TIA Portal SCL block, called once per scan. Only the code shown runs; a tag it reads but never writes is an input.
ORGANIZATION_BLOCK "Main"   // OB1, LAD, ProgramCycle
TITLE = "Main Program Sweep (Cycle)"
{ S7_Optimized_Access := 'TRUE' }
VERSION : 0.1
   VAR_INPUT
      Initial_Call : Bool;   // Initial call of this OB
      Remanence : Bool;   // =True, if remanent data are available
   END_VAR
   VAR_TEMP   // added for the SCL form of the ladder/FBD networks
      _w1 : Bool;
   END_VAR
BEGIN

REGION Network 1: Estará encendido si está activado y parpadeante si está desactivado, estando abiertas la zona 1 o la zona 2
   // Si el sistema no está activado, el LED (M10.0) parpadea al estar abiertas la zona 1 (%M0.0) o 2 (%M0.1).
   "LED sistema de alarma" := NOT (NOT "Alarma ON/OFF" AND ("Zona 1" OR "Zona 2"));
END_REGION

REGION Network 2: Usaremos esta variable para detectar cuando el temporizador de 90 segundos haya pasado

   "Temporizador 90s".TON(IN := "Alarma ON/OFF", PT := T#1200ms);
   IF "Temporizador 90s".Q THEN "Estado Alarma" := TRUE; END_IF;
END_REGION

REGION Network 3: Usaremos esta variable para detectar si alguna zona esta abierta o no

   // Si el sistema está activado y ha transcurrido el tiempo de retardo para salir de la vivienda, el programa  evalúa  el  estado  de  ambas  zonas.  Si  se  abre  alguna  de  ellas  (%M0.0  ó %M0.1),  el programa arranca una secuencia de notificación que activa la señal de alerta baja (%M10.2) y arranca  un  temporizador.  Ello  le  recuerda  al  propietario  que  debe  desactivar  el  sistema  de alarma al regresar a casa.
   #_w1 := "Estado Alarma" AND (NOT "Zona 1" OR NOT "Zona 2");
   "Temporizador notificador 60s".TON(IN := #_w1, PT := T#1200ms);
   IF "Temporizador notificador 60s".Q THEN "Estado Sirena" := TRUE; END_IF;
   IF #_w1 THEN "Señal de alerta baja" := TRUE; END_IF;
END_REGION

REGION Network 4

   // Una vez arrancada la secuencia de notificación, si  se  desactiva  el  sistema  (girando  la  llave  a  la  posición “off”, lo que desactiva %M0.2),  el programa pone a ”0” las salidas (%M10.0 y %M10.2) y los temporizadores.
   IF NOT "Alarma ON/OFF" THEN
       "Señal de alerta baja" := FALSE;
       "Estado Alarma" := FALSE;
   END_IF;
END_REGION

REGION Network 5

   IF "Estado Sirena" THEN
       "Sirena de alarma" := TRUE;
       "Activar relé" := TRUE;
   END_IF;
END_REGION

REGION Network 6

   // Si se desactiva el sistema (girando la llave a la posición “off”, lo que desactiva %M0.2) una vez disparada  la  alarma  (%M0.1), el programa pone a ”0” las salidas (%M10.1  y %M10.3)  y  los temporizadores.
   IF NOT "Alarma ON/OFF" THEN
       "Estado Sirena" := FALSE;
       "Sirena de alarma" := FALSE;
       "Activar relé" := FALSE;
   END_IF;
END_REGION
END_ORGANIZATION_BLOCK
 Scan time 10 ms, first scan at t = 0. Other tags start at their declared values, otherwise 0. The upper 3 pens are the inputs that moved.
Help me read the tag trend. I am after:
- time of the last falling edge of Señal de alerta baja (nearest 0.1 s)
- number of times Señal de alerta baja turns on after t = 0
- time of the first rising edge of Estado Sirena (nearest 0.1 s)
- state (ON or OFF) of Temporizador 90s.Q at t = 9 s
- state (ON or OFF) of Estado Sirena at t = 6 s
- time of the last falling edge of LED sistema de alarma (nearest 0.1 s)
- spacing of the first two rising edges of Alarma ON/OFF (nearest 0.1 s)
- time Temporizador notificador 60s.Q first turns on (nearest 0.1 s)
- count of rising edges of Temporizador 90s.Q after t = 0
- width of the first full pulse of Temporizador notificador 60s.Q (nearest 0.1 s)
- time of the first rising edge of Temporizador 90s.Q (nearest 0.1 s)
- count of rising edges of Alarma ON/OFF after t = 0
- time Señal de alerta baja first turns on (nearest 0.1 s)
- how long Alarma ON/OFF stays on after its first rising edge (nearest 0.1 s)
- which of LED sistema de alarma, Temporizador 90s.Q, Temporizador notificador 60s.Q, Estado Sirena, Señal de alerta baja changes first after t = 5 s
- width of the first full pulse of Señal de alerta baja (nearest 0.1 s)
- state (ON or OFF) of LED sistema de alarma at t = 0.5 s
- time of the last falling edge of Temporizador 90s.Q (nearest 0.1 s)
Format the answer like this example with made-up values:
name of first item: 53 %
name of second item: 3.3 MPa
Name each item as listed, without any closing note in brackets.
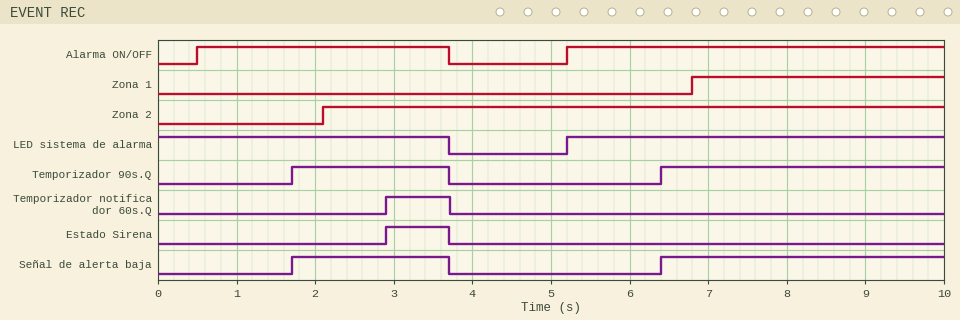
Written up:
time of the last falling edge of Señal de alerta baja: 3.7 s
number of times Señal de alerta baja turns on after t = 0: 2
time of the first rising edge of Estado Sirena: 2.9 s
state (ON or OFF) of Temporizador 90s.Q at t = 9 s: ON
state (ON or OFF) of Estado Sirena at t = 6 s: OFF
time of the last falling edge of LED sistema de alarma: 3.7 s
spacing of the first two rising edges of Alarma ON/OFF: 4.7 s
time Temporizador notificador 60s.Q first turns on: 2.9 s
count of rising edges of Temporizador 90s.Q after t = 0: 2
width of the first full pulse of Temporizador notificador 60s.Q: 0.8 s
time of the first rising edge of Temporizador 90s.Q: 1.7 s
count of rising edges of Alarma ON/OFF after t = 0: 2
time Señal de alerta baja first turns on: 1.7 s
how long Alarma ON/OFF stays on after its first rising edge: 3.2 s
which of LED sistema de alarma, Temporizador 90s.Q, Temporizador notificador 60s.Q, Estado Sirena, Señal de alerta baja changes first after t = 5 s: LED sistema de alarma
width of the first full pulse of Señal de alerta baja: 2.0 s
state (ON or OFF) of LED sistema de alarma at t = 0.5 s: ON
time of the last falling edge of Temporizador 90s.Q: 3.7 s
